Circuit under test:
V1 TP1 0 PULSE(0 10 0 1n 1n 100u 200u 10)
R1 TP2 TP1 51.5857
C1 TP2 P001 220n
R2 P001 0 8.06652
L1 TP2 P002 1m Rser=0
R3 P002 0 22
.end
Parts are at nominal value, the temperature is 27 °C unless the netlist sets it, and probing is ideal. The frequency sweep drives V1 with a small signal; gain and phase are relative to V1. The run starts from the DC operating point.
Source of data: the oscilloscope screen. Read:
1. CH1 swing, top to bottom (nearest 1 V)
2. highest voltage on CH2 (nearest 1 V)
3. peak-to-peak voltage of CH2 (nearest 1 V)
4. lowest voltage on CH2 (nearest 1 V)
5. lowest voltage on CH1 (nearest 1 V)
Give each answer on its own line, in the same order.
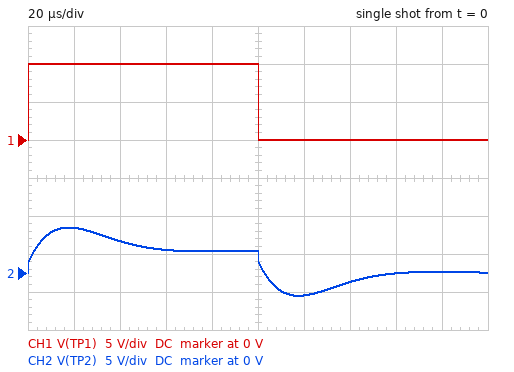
10 V
6 V
9 V
-3 V
0 V
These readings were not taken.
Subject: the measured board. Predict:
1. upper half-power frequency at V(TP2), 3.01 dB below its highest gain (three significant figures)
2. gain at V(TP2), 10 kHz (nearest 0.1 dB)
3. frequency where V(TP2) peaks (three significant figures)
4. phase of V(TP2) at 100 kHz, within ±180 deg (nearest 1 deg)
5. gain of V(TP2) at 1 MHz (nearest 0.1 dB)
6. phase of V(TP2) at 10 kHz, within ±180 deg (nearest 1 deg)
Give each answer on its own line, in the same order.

22.7 kHz
-2.5 dB
11.5 kHz
-34 deg
-17.3 dB
1 deg
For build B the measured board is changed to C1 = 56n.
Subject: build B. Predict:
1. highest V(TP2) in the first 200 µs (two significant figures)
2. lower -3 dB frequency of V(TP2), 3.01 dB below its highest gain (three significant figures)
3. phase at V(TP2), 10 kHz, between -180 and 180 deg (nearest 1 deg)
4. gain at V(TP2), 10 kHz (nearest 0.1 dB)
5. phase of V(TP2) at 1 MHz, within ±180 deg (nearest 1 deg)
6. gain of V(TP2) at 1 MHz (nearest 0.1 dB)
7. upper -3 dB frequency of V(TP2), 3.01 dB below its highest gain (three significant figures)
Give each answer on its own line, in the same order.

7.7 V
8.22 kHz
24 deg
-2.8 dB
-17 deg
-16.9 dB
61.7 kHz
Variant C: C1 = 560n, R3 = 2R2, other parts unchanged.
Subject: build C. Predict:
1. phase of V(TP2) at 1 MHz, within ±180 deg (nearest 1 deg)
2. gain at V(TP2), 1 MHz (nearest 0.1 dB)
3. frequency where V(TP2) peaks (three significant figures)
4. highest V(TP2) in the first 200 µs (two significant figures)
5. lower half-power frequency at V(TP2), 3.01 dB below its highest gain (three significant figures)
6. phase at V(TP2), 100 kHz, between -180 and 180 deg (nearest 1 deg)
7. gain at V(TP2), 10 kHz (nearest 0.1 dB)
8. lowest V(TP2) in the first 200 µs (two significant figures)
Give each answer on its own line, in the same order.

-2 deg
-17.4 dB
6.43 kHz
4.4 V
4.02 kHz
-16 deg
-4.8 dB
-4.6 V
